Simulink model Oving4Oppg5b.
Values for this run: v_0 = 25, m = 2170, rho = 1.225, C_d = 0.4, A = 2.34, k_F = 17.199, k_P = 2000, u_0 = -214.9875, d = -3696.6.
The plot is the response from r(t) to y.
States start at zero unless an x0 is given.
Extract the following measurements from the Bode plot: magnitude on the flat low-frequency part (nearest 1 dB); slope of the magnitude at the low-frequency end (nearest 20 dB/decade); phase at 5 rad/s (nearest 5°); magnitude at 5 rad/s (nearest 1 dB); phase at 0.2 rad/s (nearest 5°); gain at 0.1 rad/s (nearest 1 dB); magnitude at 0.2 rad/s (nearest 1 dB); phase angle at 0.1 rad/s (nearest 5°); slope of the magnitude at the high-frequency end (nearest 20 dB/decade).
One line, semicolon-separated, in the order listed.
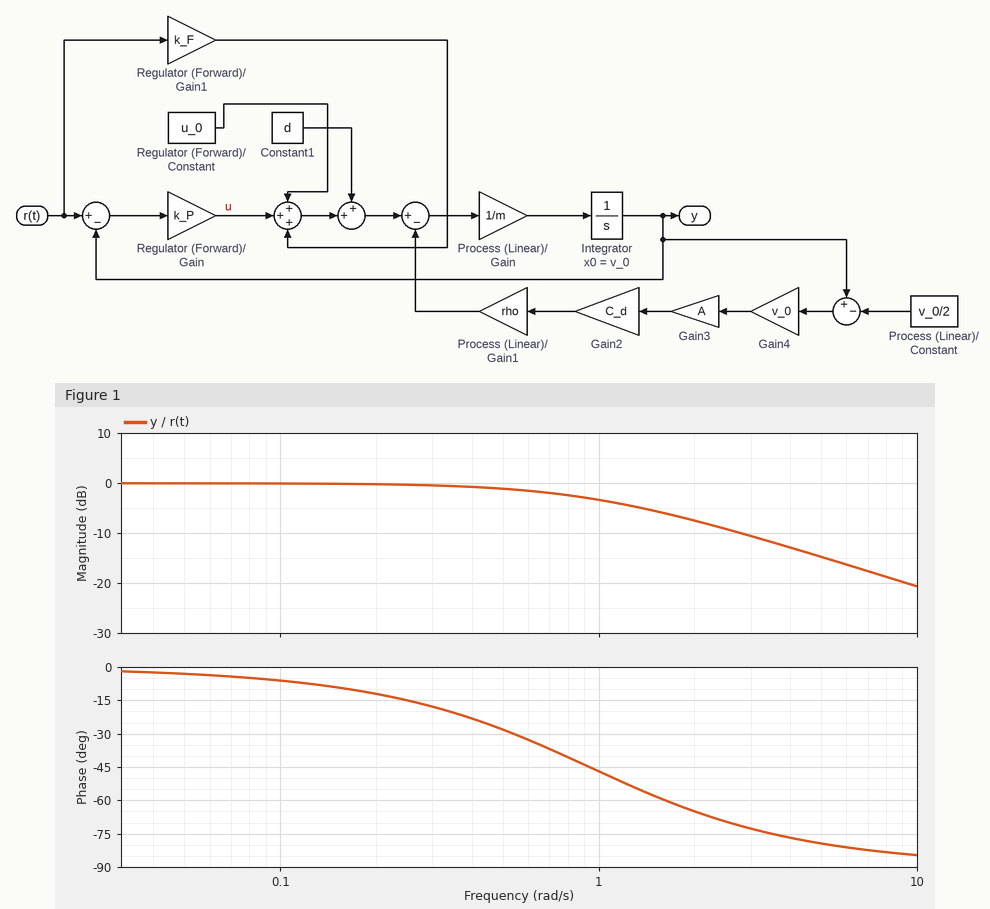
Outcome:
0 dB; 0 dB/decade; -80°; -15 dB; -10°; 0 dB; 0 dB; -5°; -20 dB/decade
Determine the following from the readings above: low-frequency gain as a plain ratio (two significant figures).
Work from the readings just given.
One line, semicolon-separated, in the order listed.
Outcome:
1.0
